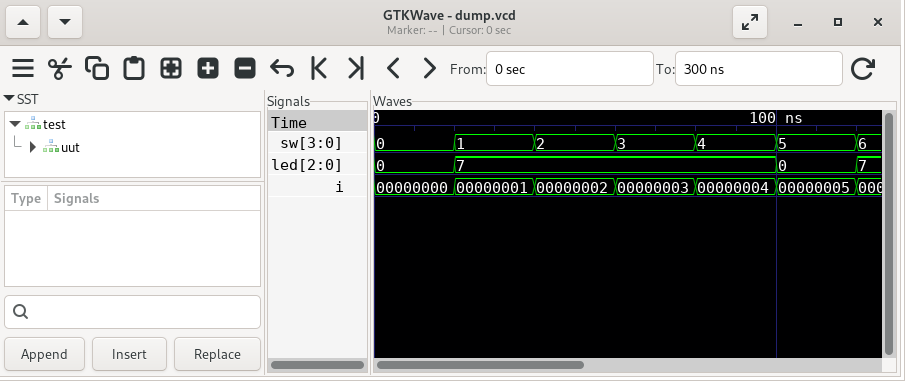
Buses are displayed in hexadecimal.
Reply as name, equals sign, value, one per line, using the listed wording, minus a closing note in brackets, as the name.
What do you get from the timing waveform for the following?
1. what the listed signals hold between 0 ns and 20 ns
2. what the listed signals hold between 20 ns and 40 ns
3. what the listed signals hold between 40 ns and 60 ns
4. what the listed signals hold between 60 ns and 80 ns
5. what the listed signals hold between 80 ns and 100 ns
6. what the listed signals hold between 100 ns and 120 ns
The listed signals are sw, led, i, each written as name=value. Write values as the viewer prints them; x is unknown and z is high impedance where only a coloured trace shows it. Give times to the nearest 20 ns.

what the listed signals hold between 0 ns and 20 ns = sw=0, led=0, i=00000000
what the listed signals hold between 20 ns and 40 ns = sw=1, led=7, i=00000001
what the listed signals hold between 40 ns and 60 ns = sw=2, led=7, i=00000002
what the listed signals hold between 60 ns and 80 ns = sw=3, led=7, i=00000003
what the listed signals hold between 80 ns and 100 ns = sw=4, led=7, i=00000004
what the listed signals hold between 100 ns and 120 ns = sw=5, led=0, i=00000005
